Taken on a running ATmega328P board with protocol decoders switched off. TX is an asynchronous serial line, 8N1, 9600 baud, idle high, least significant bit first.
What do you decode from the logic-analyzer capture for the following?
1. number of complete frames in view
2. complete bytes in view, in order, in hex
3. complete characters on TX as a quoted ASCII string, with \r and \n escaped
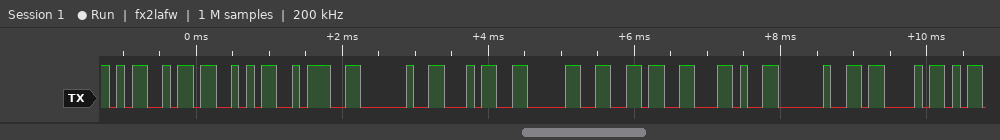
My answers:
10
0x4D 0x53 0x3A 0x20 0x34 0x30 0x36 0x2C 0x20 0x43
"MS: 406, C"
